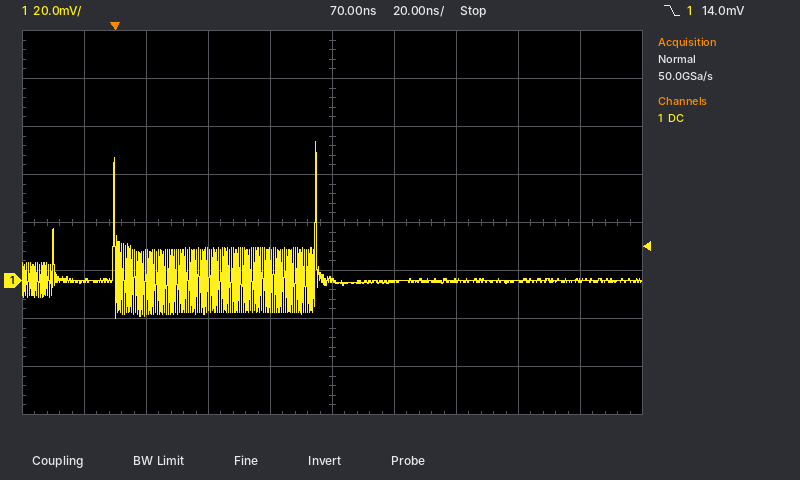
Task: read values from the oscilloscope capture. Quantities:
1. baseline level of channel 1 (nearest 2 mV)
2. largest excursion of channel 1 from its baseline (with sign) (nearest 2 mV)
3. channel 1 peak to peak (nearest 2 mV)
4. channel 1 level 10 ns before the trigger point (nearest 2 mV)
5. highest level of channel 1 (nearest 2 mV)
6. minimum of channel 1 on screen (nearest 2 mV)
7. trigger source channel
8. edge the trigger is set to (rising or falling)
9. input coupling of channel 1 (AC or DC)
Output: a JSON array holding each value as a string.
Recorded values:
["0 mV", "+58 mV", "74 mV", "0 mV", "58 mV", "-16 mV", "channel 1", "falling", "DC"]
